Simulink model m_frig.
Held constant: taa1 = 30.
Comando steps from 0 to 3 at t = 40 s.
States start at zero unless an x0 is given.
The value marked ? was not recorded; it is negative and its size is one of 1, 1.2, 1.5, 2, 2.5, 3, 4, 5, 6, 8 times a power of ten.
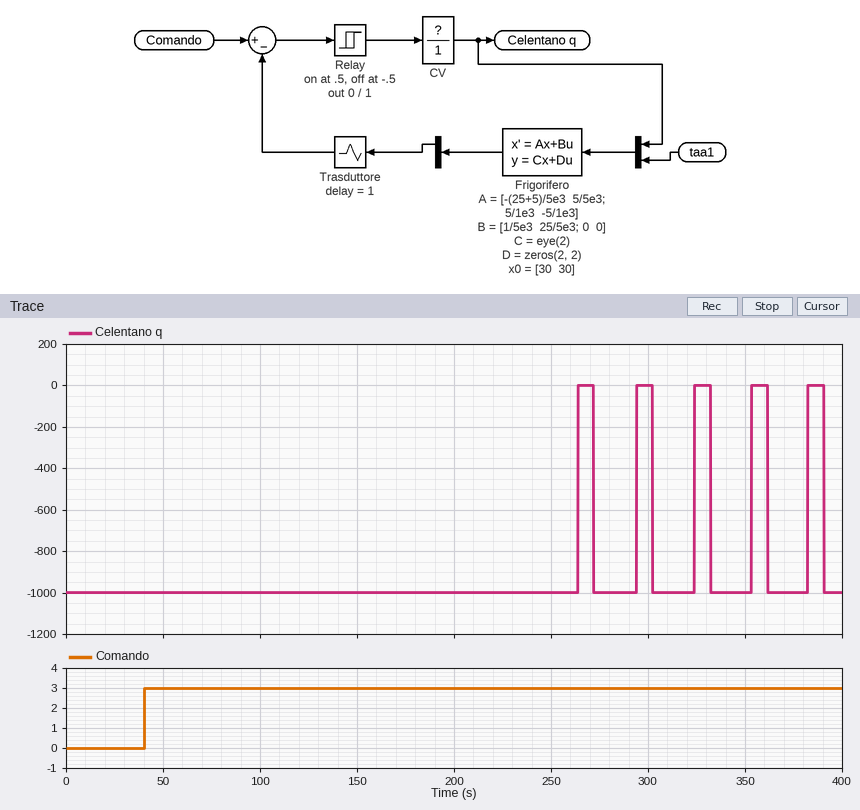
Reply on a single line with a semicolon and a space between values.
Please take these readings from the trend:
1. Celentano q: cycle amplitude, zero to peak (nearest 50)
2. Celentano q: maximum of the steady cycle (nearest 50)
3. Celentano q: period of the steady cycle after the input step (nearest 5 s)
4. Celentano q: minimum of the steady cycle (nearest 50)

500; 0; 30 s; -1000
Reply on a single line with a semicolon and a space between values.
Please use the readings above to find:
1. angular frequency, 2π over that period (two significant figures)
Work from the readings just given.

0.21 rad/s
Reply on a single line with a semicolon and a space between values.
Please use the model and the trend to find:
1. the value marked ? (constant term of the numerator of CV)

-1000
